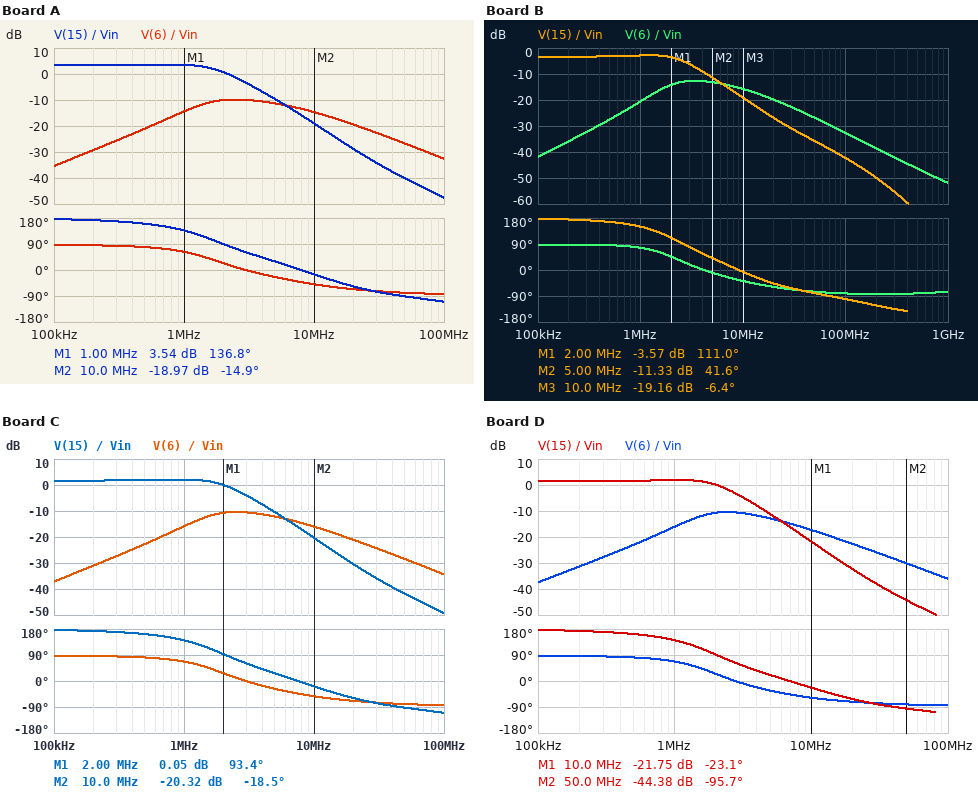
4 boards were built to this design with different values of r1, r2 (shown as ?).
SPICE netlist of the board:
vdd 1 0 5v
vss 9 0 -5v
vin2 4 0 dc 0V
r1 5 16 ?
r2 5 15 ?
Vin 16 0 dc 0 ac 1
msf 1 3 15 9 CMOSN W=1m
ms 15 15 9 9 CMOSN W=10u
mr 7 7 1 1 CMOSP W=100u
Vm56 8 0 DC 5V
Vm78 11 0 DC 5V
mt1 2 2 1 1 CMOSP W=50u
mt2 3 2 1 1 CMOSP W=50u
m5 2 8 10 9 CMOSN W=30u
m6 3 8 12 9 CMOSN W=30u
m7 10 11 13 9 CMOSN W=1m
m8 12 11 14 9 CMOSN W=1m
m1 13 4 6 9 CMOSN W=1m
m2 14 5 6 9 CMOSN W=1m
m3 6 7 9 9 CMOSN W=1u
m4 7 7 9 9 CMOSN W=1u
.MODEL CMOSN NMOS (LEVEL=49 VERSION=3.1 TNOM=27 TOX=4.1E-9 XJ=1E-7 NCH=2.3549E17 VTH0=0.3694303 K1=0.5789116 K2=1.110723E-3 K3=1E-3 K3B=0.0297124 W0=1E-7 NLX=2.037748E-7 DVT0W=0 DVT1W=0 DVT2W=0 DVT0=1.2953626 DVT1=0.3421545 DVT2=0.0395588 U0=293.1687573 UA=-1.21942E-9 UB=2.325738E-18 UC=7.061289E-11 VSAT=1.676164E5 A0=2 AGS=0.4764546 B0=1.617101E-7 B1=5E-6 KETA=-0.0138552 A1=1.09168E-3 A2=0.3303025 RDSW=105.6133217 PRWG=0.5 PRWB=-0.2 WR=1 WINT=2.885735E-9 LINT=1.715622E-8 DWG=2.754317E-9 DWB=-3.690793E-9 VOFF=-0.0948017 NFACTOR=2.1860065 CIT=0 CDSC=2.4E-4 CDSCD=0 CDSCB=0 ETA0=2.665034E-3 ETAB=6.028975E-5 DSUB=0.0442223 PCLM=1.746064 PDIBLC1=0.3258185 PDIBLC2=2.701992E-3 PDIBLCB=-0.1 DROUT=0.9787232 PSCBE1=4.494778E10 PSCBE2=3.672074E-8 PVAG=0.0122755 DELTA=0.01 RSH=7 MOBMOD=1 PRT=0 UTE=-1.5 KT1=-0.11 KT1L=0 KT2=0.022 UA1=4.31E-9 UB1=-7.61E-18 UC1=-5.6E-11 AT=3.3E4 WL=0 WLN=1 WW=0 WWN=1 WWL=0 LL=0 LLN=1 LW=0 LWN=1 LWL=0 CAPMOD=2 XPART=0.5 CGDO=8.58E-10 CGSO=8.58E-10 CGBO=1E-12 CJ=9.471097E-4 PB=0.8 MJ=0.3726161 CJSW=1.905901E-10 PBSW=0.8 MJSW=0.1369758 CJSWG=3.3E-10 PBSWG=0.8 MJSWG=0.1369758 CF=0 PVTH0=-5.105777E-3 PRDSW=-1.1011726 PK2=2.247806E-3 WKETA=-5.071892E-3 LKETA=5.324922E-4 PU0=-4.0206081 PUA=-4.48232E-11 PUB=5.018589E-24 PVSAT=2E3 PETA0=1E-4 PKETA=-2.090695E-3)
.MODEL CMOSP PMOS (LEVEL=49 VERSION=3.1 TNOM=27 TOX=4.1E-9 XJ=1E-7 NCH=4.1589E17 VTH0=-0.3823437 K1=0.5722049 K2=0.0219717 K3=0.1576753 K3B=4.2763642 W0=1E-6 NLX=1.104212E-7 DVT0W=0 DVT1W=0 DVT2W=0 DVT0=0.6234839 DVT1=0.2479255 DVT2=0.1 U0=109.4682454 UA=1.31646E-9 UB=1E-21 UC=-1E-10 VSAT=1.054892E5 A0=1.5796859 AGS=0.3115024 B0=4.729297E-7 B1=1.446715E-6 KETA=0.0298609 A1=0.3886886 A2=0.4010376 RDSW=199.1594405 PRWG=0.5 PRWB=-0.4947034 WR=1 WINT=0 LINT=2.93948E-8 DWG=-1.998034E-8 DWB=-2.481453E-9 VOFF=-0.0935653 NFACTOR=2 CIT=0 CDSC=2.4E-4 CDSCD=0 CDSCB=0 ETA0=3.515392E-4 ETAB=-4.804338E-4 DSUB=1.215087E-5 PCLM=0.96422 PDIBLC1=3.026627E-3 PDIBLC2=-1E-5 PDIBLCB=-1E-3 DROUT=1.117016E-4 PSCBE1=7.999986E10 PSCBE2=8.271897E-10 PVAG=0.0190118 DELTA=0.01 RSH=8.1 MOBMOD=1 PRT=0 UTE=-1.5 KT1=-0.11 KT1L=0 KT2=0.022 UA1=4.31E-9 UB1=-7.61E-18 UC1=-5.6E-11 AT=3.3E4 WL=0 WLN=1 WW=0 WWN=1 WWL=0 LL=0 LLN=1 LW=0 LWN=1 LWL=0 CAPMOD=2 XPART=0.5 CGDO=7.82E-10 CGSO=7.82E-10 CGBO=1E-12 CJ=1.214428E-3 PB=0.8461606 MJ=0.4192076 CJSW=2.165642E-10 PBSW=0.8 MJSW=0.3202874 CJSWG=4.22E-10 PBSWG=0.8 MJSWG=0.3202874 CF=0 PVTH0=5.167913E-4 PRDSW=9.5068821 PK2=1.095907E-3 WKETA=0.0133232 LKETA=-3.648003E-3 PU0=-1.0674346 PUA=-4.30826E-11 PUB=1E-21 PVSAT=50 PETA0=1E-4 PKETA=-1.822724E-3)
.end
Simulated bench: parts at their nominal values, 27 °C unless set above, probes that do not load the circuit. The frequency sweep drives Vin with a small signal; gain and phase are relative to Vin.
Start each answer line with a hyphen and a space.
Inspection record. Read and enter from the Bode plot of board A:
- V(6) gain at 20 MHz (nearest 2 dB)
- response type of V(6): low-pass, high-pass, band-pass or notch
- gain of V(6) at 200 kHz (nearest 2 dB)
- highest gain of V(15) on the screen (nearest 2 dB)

- -20 dB
- band-pass
- -30 dB
- 4 dB
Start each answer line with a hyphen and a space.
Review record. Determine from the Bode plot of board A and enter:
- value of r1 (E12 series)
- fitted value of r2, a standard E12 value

- 2.2 kΩ
- 3.3 kΩ
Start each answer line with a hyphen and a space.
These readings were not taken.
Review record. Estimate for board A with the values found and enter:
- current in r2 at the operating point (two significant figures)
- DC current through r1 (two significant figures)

- 2.1 µA
- 2.1 µA
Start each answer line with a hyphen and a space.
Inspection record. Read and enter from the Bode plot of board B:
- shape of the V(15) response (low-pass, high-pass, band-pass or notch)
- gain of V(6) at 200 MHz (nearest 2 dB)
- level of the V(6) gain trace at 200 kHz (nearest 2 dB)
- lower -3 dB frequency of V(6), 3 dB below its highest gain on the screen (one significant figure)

- low-pass
- -38 dB
- -36 dB
- 2 MHz
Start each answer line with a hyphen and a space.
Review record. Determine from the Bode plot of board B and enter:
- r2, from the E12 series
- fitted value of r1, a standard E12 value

- 1.5 kΩ
- 2.2 kΩ
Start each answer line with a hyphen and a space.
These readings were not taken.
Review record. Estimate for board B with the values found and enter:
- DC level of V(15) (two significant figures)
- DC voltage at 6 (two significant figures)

- 7.9 mV
- -1.1 V
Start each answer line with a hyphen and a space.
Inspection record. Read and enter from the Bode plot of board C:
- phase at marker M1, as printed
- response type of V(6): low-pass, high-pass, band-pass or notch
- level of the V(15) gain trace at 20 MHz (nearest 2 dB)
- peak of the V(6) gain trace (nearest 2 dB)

- 93.4 deg
- band-pass
- -30 dB
- -10 dB
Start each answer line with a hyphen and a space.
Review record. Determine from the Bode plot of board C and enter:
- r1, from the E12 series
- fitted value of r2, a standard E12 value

- 2.7 kΩ
- 3.3 kΩ
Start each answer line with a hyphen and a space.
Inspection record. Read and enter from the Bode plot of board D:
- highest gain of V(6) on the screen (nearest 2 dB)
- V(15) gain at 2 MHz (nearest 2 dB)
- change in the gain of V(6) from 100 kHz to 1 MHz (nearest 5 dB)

- -10 dB
- 0 dB
- 20 dB
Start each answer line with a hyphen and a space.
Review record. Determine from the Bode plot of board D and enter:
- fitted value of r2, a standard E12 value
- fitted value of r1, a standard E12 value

- 3.9 kΩ
- 3.3 kΩ
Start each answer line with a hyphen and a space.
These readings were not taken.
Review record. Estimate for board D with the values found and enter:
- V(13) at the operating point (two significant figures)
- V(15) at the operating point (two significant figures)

- 3.1 V
- 10 mV
